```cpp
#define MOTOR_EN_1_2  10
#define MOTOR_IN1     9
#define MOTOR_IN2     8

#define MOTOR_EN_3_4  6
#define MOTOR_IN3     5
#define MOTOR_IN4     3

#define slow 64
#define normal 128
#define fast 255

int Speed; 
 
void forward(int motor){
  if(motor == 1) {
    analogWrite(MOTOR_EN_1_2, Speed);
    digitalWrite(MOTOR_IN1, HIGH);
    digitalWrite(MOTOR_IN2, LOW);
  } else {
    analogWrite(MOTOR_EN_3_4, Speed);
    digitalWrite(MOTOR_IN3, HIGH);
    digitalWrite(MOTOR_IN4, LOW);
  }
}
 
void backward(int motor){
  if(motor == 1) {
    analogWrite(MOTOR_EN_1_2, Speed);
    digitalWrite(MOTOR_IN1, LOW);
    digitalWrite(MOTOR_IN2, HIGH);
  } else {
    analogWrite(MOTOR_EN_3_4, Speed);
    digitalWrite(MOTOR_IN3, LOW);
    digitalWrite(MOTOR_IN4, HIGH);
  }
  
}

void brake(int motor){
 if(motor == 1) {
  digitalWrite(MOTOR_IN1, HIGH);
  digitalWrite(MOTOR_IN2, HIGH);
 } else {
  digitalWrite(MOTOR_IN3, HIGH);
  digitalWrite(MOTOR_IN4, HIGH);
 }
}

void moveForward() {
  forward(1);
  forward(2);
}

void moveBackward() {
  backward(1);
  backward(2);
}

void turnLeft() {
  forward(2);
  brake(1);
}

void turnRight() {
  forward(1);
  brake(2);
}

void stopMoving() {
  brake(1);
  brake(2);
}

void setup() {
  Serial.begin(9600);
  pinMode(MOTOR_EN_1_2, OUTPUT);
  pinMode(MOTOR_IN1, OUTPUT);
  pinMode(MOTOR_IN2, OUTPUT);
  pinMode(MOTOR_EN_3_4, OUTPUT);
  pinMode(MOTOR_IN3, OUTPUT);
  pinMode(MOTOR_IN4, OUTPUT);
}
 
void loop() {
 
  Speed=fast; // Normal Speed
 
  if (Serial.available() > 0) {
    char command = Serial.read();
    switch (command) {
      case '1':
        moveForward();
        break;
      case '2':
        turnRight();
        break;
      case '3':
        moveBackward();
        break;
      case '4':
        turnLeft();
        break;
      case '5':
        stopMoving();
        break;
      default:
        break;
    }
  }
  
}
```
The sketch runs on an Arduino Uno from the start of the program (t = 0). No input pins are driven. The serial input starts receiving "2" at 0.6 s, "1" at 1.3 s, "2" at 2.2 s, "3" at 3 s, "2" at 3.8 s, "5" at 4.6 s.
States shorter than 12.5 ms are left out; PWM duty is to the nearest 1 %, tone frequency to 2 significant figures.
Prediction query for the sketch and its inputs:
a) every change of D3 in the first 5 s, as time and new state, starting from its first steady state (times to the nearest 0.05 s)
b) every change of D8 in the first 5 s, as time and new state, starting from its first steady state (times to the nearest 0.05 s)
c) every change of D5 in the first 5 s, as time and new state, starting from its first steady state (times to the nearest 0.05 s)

0 s low; 0.6 s high; 1.3 s low; 2.2 s high
0 s low; 3 s high; 3.8 s low; 4.6 s high
0 s low; 0.6 s high; 3 s low; 3.8 s high
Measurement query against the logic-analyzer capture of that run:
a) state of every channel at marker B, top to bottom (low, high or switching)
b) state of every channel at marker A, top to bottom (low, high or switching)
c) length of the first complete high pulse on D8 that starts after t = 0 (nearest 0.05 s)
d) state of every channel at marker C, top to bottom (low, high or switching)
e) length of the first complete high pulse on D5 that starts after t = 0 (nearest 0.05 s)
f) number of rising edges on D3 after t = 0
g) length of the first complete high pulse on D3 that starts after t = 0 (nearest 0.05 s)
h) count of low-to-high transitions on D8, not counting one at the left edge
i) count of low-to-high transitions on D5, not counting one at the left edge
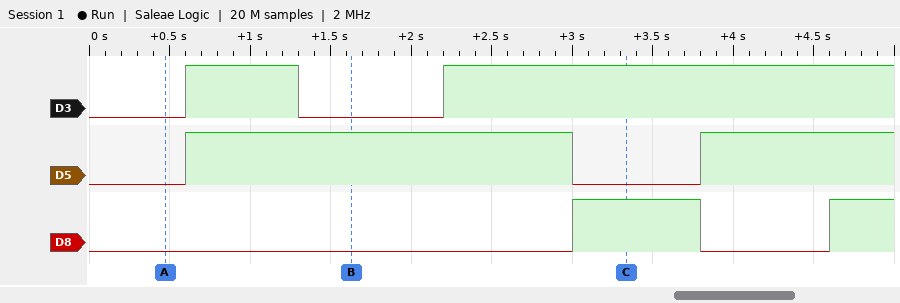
D3 low, D5 high, D8 low
D3 low, D5 low, D8 low
0.80 s
D3 high, D5 low, D8 high
2.40 s
2
0.70 s
2
2
